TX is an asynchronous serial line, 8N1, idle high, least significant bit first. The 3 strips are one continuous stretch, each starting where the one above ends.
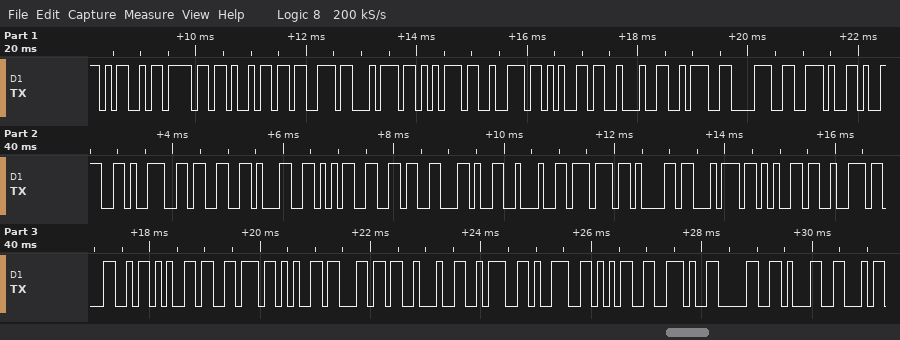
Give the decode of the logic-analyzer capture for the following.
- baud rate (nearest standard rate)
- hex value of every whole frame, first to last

9600 baud
4D 6F 69 73 74 75 72 65 22 3A 38 2E 39 39 33 31 35 36 2C 22 77 61 74 65 72 4C 65 76 65 6C 22 3A 39 35 2E 30 31
